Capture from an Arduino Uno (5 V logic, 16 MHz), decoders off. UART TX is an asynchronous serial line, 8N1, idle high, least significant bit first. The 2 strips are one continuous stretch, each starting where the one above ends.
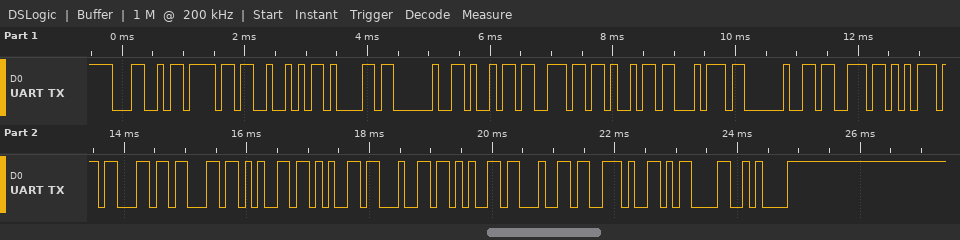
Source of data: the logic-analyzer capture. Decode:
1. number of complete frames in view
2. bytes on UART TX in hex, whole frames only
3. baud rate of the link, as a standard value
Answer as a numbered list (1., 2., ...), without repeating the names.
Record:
1. 22
2. 4C 6F 52 61 20 69 6E 69 74 20 73 75 63 63 65 65 64 65 64 2E 0D 0A
3. 9600 baud
